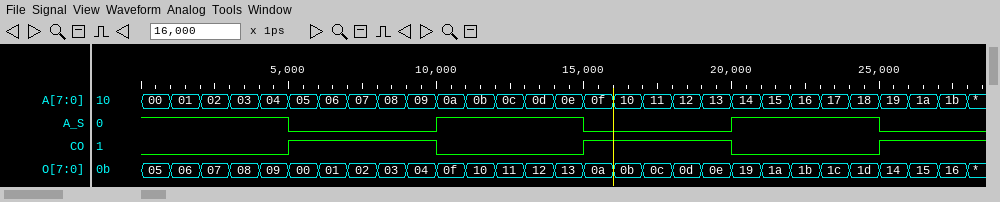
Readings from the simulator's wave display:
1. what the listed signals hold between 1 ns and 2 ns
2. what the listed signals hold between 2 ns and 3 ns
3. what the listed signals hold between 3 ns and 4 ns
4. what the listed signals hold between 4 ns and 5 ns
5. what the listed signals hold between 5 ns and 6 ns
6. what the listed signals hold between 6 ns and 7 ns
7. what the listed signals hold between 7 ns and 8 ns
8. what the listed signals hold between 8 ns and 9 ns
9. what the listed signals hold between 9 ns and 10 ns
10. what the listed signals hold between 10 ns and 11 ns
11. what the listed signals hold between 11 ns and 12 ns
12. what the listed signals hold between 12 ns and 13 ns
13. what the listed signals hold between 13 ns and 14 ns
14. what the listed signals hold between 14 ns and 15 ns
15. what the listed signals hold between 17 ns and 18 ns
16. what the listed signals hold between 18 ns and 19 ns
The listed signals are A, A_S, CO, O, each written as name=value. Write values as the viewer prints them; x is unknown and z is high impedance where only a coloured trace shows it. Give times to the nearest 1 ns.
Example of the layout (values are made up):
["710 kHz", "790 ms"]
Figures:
["A=01, A_S=1, CO=0, O=06", "A=02, A_S=1, CO=0, O=07", "A=03, A_S=1, CO=0, O=08", "A=04, A_S=1, CO=0, O=09", "A=05, A_S=0, CO=1, O=00", "A=06, A_S=0, CO=1, O=01", "A=07, A_S=0, CO=1, O=02", "A=08, A_S=0, CO=1, O=03", "A=09, A_S=0, CO=1, O=04", "A=0a, A_S=1, CO=0, O=0f", "A=0b, A_S=1, CO=0, O=10", "A=0c, A_S=1, CO=0, O=11", "A=0d, A_S=1, CO=0, O=12", "A=0e, A_S=1, CO=0, O=13", "A=11, A_S=0, CO=1, O=0c", "A=12, A_S=0, CO=1, O=0d"]
